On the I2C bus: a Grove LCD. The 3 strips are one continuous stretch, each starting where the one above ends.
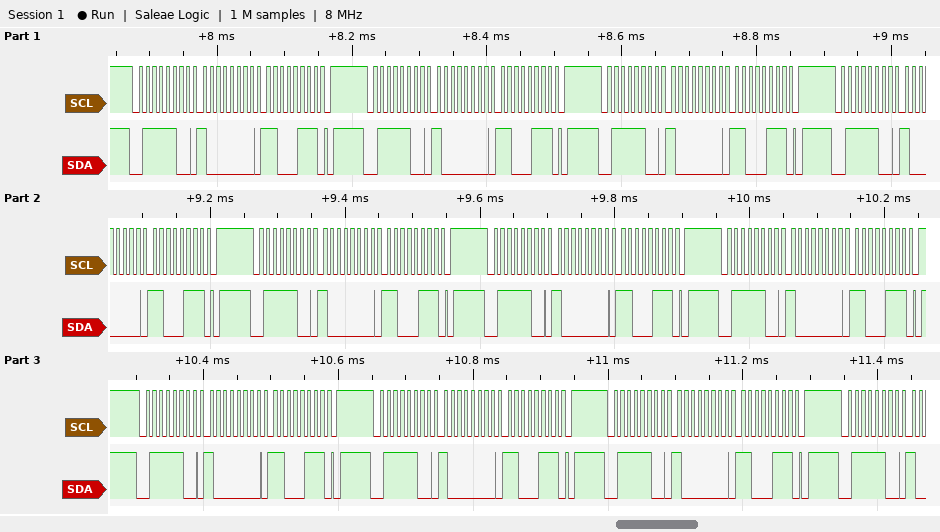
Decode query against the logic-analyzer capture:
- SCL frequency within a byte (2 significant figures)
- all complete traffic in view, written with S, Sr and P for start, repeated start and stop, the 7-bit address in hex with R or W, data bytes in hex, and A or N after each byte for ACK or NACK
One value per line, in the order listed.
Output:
100 kHz
S 3EW A 80 A C7 A P S 3EW A 80 A C7 A P S 3EW A 80 A C7 A P S 3EW A 80 A C7 A P S 3EW A 80 A C7 A P S 3EW A 80 A C7 A P S 3EW A 80 A C7 A P S 3EW A 80 A C7 A P S 3EW A 80 A C7 A P S 3EW A 80 A C7 A P S 3EW A
